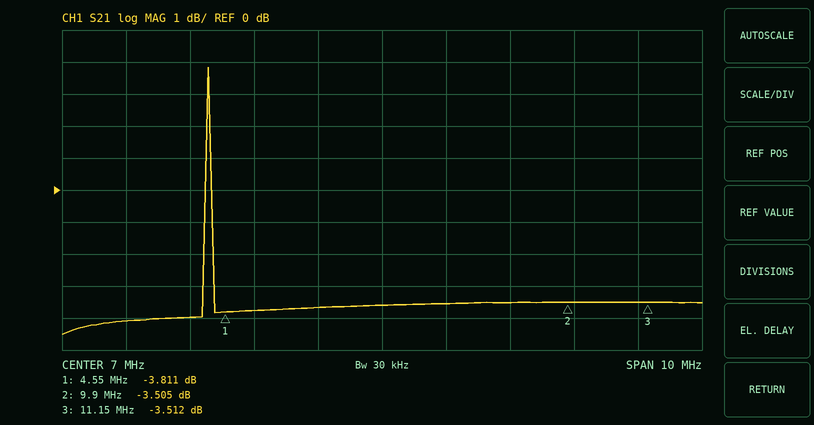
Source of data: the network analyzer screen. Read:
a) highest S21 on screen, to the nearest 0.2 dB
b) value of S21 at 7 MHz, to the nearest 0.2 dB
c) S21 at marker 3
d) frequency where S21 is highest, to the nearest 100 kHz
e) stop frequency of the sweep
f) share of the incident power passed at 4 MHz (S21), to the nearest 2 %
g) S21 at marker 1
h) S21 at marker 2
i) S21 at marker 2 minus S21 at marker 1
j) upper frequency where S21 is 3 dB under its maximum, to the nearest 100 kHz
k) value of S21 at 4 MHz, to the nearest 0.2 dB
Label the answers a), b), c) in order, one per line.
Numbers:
a) 3.8 dB
b) -3.6 dB
c) -3.512 dB
d) 4.3 MHz
e) 12 MHz
f) 40 %
g) -3.811 dB
h) -3.505 dB
i) 0.306 dB
j) 4.3 MHz
k) -4.0 dB
